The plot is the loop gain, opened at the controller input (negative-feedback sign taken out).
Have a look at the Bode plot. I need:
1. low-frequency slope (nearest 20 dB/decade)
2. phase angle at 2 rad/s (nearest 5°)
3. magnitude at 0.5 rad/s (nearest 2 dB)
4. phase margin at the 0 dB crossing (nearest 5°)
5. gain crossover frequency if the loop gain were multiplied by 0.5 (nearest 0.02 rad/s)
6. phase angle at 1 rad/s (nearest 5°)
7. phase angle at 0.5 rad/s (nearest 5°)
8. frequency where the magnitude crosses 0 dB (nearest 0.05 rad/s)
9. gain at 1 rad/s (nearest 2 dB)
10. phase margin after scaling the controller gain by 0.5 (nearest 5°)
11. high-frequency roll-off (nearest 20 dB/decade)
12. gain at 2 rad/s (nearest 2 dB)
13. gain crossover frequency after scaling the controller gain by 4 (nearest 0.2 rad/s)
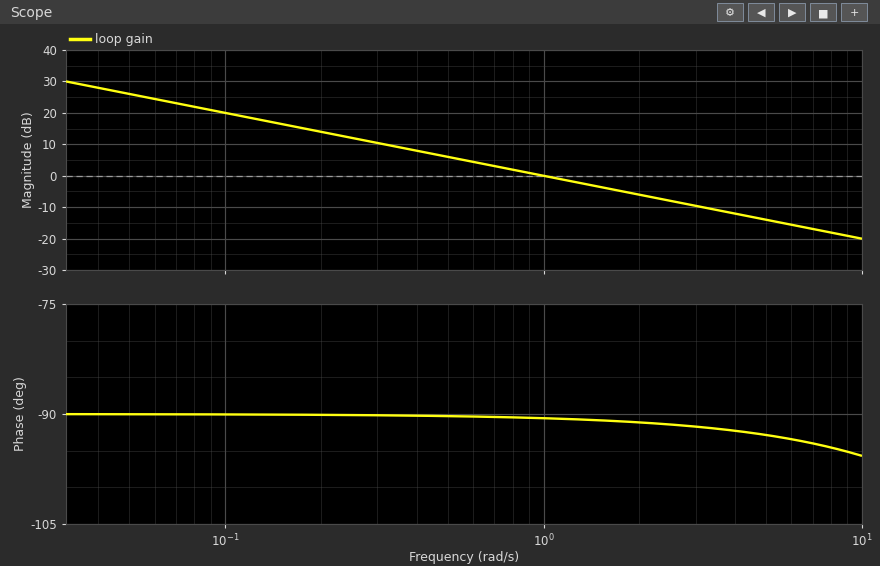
-20 dB/decade
-90°
6 dB
90°
0.50 rad/s
-90°
-90°
1.00 rad/s
0 dB
90°
-20 dB/decade
-6 dB
4.0 rad/s
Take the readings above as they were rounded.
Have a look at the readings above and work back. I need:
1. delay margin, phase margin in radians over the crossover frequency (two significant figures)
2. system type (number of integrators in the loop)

1.6 s
1
